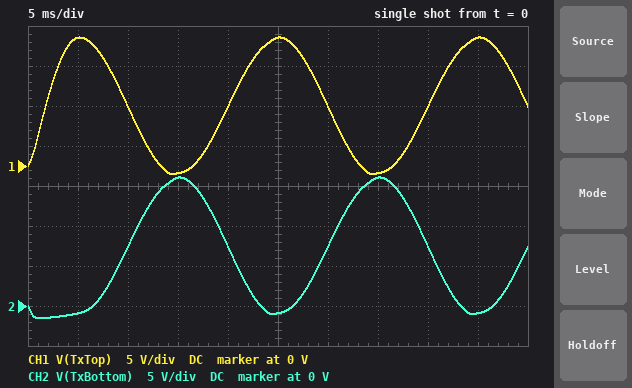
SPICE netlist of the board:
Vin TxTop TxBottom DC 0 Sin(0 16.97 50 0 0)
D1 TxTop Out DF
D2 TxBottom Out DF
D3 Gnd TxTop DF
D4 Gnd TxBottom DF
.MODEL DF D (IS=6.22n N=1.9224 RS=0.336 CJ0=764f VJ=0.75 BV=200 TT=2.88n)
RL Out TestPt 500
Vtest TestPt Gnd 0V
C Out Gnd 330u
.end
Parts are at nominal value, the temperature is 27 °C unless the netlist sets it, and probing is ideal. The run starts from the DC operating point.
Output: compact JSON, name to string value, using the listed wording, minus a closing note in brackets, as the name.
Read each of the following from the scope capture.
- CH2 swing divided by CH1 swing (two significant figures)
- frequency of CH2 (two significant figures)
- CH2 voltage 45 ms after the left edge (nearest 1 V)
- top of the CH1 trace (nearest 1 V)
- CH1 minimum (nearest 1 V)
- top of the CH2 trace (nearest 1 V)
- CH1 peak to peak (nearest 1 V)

{"CH2 swing divided by CH1 swing": "1.0", "frequency of CH2": "50 Hz", "CH2 voltage 45 ms after the left edge": "-1 V", "top of the CH1 trace": "16 V", "CH1 minimum": "-1 V", "top of the CH2 trace": "16 V", "CH1 peak to peak": "17 V"}
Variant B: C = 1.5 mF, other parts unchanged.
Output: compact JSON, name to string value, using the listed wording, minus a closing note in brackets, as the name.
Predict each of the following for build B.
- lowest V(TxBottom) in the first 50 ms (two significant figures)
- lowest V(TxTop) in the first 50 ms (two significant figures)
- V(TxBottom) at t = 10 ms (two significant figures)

{"lowest V(TxBottom) in the first 50 ms": "-3.0 V", "lowest V(TxTop) in the first 50 ms": "-1.2 V", "V(TxBottom) at t = 10 ms": "7.1 V"}
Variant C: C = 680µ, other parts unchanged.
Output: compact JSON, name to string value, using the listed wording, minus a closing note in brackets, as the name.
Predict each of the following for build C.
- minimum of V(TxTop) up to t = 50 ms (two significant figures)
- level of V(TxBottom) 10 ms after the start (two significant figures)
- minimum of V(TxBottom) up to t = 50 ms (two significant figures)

{"minimum of V(TxTop) up to t = 50 ms": "-1.0 V", "level of V(TxBottom) 10 ms after the start": "7.4 V", "minimum of V(TxBottom) up to t = 50 ms": "-2.0 V"}
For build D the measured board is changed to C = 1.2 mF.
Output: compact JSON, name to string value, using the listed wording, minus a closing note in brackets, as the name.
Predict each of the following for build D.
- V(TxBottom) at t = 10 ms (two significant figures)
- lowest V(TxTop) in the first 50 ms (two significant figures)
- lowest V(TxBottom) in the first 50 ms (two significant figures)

{"V(TxBottom) at t = 10 ms": "7.2 V", "lowest V(TxTop) in the first 50 ms": "-1.1 V", "lowest V(TxBottom) in the first 50 ms": "-2.7 V"}
